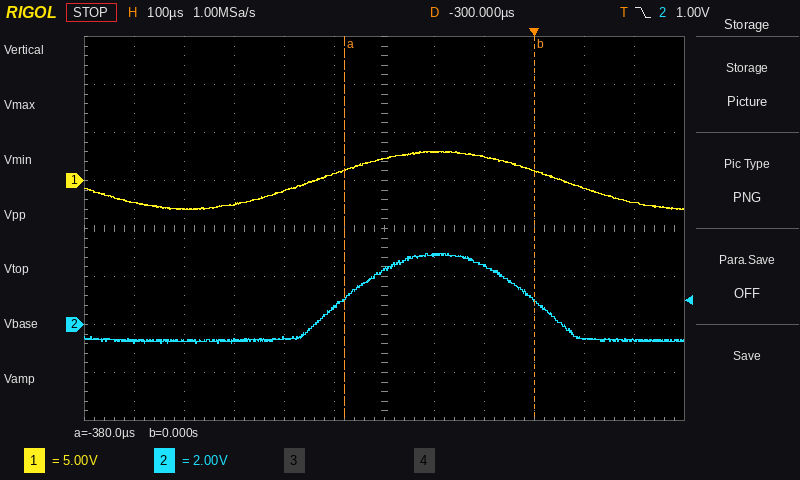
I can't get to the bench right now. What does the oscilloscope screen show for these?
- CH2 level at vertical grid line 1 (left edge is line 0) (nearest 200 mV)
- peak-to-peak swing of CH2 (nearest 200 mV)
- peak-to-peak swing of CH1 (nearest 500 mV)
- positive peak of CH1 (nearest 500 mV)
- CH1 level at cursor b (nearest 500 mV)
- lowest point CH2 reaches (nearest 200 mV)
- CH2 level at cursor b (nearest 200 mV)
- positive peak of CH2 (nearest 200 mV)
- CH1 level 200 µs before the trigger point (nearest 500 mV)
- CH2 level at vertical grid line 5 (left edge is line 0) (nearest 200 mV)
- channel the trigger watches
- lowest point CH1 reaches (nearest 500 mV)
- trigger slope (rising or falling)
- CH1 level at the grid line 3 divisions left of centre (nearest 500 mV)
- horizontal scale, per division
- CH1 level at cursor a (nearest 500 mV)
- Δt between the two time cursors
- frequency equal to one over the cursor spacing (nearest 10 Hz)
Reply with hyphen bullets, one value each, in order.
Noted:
- -800 mV
- 3.8 V
- 6.0 V
- 3.0 V
- 1.0 V
- -800 mV
- 1.0 V
- 3.0 V
- 3.0 V
- 800 mV
- CH2
- -3.0 V
- falling
- -2.5 V
- 100 µs
- 1.0 V
- 380 µs
- 2.63 kHz
